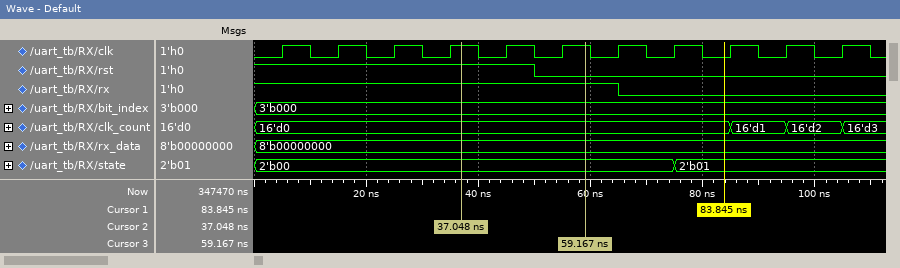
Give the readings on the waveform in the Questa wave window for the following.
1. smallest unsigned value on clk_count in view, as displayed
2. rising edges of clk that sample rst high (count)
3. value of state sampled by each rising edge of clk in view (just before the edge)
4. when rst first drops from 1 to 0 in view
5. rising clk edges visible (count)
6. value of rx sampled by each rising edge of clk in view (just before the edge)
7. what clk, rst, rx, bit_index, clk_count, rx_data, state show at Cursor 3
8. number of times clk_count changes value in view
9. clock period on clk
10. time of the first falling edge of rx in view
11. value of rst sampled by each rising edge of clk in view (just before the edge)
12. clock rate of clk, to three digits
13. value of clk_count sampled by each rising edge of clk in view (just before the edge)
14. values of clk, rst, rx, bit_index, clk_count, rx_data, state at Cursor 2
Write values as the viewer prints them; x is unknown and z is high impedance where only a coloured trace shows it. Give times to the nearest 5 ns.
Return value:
16'd0
5
2'b00, 2'b00, 2'b00, 2'b00, 2'b00, 2'b00, 2'b00, 2'b00, 2'b01, 2'b01, 2'b01
50 ns
11
1 1 1 1 1 1 1 0 0 0 0
clk=1, rst=0, rx=1, bit_index=3'b000, clk_count=16'd0, rx_data=8'b00000000, state=2'b00
3
10 ns
65 ns
1 1 1 1 1 0 0 0 0 0 0
100 MHz
16'd0, 16'd0, 16'd0, 16'd0, 16'd0, 16'd0, 16'd0, 16'd0, 16'd0, 16'd1, 16'd2
clk=1, rst=1, rx=1, bit_index=3'b000, clk_count=16'd0, rx_data=8'b00000000, state=2'b00
